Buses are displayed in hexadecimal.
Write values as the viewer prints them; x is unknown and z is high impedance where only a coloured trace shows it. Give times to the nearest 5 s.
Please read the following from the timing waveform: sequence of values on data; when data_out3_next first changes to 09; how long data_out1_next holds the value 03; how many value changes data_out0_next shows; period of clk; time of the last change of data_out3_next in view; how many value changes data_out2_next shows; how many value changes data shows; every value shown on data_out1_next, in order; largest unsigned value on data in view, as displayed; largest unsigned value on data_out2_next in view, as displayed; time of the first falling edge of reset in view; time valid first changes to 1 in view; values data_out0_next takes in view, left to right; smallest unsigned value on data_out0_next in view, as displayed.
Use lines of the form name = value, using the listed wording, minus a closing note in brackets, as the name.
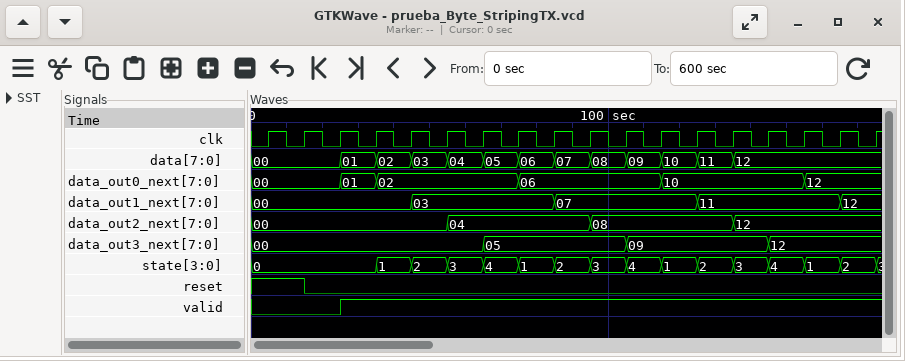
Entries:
sequence of values on data = 00, 01, 02, 03, 04, 05, 06, 07, 08, 09, 10, 11, 12
when data_out3_next first changes to 09 = 105 s
how long data_out1_next holds the value 03 = 40 s
how many value changes data_out0_next shows = 5
period of clk = 10 s
time of the last change of data_out3_next in view = 145 s
how many value changes data_out2_next shows = 3
how many value changes data shows = 12
every value shown on data_out1_next, in order = 00, 03, 07, 11, 12
largest unsigned value on data in view, as displayed = 12
largest unsigned value on data_out2_next in view, as displayed = 12
time of the first falling edge of reset in view = 15 s
time valid first changes to 1 in view = 25 s
values data_out0_next takes in view, left to right = 00, 01, 02, 06, 10, 12
smallest unsigned value on data_out0_next in view, as displayed = 00
